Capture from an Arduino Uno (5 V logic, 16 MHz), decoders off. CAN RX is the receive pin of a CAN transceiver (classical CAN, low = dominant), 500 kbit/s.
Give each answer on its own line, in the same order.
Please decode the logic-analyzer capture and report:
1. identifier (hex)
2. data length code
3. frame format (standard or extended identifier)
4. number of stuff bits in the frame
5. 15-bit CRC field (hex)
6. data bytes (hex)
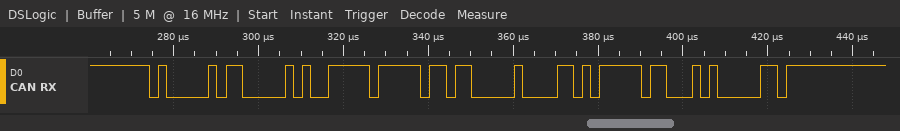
0x40C
4
standard
7
0x78A0
FF F6 00 D7
